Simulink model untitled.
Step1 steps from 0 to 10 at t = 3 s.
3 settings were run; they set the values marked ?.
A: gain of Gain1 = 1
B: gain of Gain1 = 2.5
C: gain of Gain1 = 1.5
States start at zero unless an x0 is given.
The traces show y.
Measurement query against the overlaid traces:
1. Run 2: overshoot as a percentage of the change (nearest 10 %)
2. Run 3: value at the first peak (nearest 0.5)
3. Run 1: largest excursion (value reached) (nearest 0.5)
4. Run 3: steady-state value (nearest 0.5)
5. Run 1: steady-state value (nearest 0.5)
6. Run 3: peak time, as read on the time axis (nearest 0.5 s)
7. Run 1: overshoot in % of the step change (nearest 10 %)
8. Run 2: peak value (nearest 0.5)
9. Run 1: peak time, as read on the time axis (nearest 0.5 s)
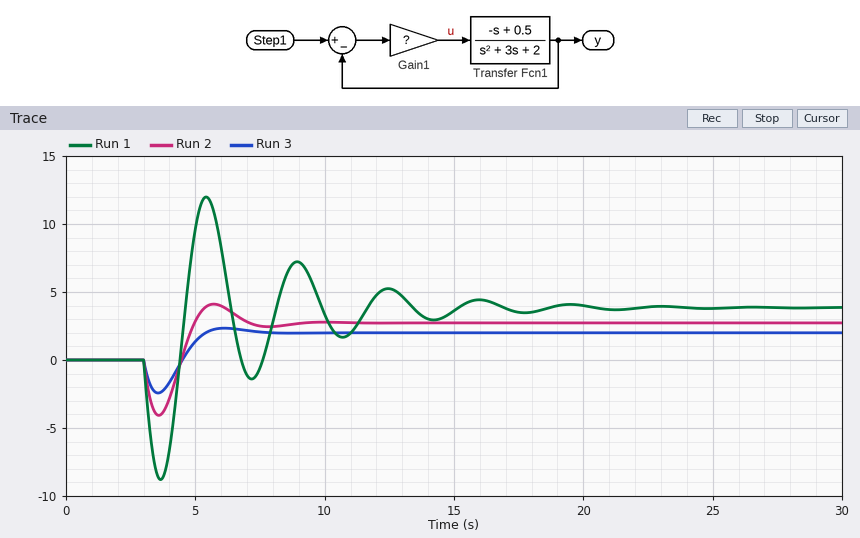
50 %
2.5
12.0
2.0
4.0
6.0 s
210 %
4.0
5.5 s
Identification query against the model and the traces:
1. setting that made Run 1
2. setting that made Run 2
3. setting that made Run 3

B
C
A
